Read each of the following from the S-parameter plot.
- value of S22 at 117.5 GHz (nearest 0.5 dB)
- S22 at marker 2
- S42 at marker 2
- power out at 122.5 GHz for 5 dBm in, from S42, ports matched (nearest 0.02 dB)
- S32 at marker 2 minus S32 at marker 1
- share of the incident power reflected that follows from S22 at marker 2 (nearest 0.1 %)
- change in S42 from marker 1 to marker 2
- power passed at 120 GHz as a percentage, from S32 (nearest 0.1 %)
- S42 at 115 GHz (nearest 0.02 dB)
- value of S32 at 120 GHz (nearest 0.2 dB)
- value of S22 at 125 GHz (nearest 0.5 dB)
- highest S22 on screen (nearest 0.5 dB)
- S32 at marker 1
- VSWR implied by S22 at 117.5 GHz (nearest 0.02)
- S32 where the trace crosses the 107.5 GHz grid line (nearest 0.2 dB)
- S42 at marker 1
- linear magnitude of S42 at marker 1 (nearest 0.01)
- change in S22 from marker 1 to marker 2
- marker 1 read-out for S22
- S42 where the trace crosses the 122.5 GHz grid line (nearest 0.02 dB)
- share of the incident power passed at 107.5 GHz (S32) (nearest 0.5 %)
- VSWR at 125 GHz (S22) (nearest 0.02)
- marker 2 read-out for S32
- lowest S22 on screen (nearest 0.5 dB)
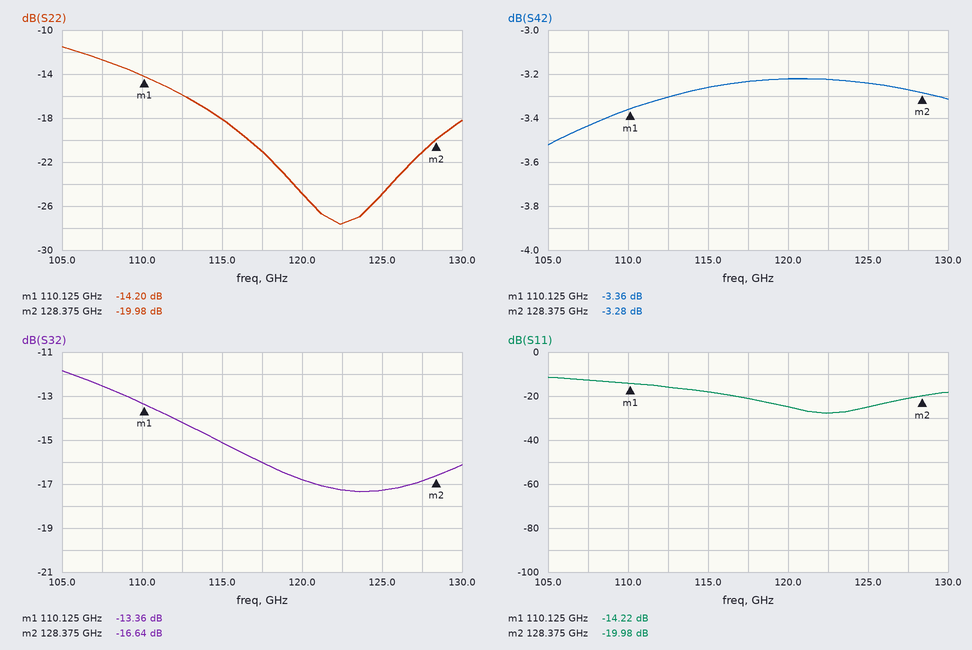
-21.0 dB
-19.98 dB
-3.28 dB
1.78 dBm
-3.28 dB
1.0 %
0.08 dB
2.1 %
-3.26 dB
-16.8 dB
-25.0 dB
-11.5 dB
-13.36 dB
1.20
-12.6 dB
-3.36 dB
0.68
-5.78 dB
-14.20 dB
-3.22 dB
5.5 %
1.12
-16.64 dB
-27.5 dB
